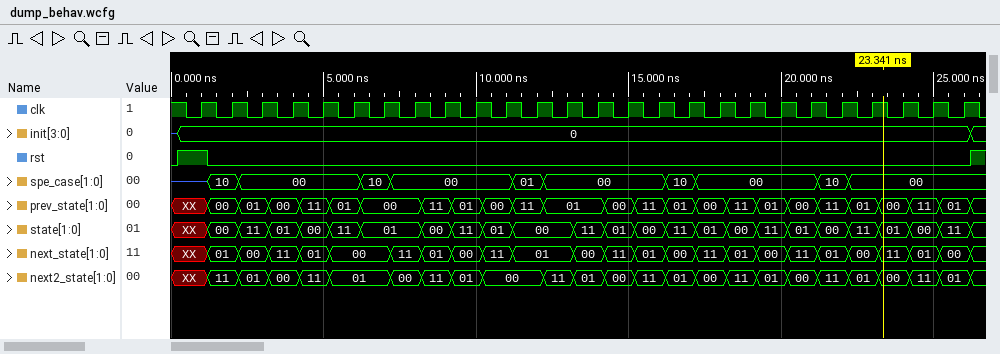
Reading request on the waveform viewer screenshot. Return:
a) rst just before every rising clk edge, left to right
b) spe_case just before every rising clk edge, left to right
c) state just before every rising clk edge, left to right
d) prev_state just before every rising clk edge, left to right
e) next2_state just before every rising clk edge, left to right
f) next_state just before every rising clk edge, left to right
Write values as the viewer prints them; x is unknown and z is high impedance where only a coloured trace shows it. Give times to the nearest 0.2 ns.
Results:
1 0 0 0 0 0 0 0 0 0 0 0 0 0 0 0 0 0 0 0 0 0 0 0 0 0
z, 10, 00, 00, 00, 00, 10, 00, 00, 00, 00, 01, 00, 00, 00, 00, 10, 00, 00, 00, 00, 10, 00, 00, 00, 00
XX, 00, 11, 01, 00, 11, 01, 01, 00, 11, 01, 00, 00, 11, 01, 00, 11, 01, 00, 11, 01, 00, 11, 01, 00, 11
XX, 00, 01, 00, 11, 01, 00, 00, 11, 01, 00, 11, 01, 01, 00, 11, 01, 00, 11, 01, 00, 11, 01, 00, 11, 01
XX, 11, 01, 00, 11, 01, 01, 00, 11, 01, 00, 00, 11, 01, 00, 11, 01, 00, 11, 01, 00, 11, 01, 00, 11, 01
XX, 01, 00, 11, 01, 00, 00, 11, 01, 00, 11, 01, 01, 00, 11, 01, 00, 11, 01, 00, 11, 01, 00, 11, 01, 00
